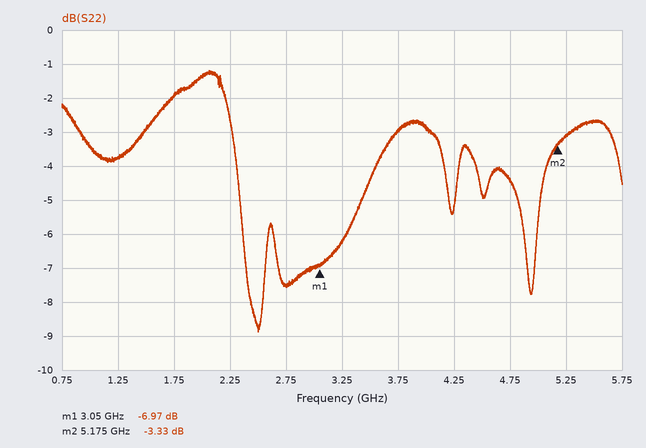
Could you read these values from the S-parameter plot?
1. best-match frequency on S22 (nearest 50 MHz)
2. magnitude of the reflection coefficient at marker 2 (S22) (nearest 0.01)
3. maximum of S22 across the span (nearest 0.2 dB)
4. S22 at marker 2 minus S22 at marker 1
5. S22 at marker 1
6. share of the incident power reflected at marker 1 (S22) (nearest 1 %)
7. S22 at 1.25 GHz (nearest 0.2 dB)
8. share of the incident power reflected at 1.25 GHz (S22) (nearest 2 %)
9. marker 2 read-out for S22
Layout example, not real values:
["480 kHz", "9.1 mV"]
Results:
["2.50 GHz", "0.68", "-1.2 dB", "3.64 dB", "-6.97 dB", "20 %", "-3.8 dB", "42 %", "-3.33 dB"]
